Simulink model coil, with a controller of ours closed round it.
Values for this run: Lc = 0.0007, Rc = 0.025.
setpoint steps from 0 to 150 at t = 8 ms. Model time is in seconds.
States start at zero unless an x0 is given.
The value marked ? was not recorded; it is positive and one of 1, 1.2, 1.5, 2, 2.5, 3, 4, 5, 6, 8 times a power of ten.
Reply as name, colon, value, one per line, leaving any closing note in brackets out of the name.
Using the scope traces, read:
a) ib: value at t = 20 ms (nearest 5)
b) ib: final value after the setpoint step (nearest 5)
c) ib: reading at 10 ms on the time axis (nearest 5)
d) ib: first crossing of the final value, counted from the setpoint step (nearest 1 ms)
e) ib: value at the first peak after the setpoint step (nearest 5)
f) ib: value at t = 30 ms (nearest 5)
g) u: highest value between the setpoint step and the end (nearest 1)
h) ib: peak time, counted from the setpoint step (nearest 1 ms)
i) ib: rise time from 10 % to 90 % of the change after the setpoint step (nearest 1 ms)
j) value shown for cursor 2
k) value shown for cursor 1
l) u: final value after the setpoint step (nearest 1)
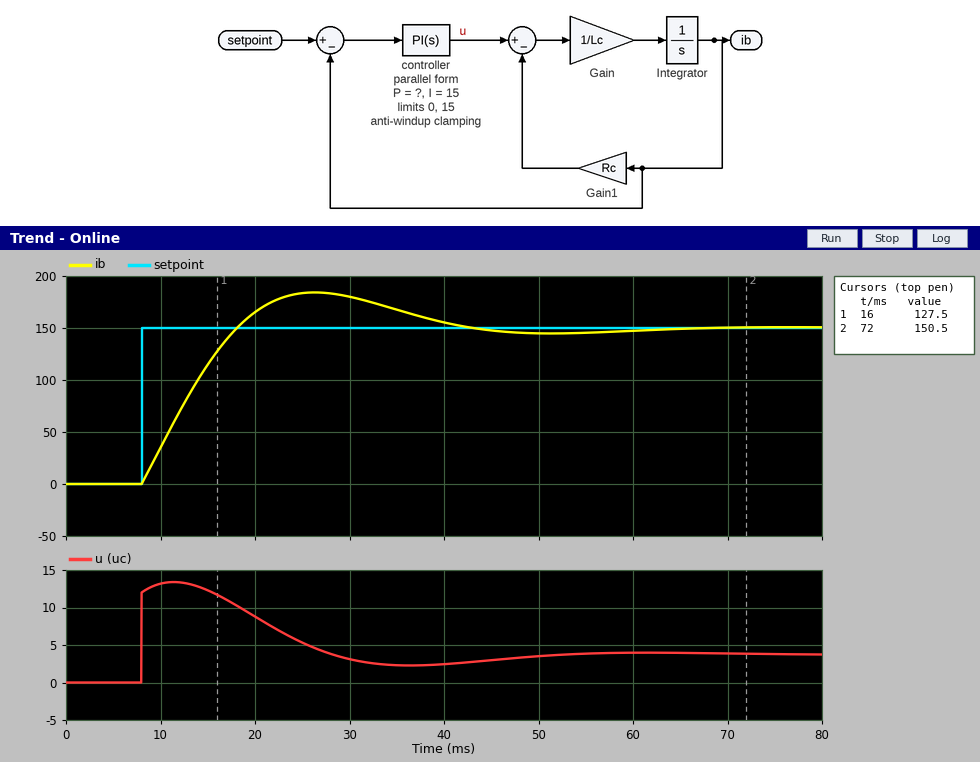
ib: value at t = 20 ms: 165
ib: final value after the setpoint step: 150
ib: reading at 10 ms on the time axis: 35
ib: first crossing of the final value, counted from the setpoint step: 10 ms
ib: value at the first peak after the setpoint step: 185
ib: value at t = 30 ms: 180
u: highest value between the setpoint step and the end: 13
ib: peak time, counted from the setpoint step: 18 ms
ib: rise time from 10 % to 90 % of the change after the setpoint step: 8 ms
value shown for cursor 2: 150.5
value shown for cursor 1: 127.5
u: final value after the setpoint step: 4
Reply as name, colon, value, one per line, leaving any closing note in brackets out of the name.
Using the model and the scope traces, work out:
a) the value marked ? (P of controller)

the value marked ?: 0.08
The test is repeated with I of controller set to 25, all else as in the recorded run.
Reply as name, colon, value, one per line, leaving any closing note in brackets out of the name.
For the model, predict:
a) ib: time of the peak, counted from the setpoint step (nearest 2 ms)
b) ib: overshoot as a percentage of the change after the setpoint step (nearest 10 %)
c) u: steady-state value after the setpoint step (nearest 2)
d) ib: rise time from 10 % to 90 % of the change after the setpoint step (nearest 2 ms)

ib: time of the peak, counted from the setpoint step: 16 ms
ib: overshoot as a percentage of the change after the setpoint step: 30 %
u: steady-state value after the setpoint step: 4
ib: rise time from 10 % to 90 % of the change after the setpoint step: 6 ms
